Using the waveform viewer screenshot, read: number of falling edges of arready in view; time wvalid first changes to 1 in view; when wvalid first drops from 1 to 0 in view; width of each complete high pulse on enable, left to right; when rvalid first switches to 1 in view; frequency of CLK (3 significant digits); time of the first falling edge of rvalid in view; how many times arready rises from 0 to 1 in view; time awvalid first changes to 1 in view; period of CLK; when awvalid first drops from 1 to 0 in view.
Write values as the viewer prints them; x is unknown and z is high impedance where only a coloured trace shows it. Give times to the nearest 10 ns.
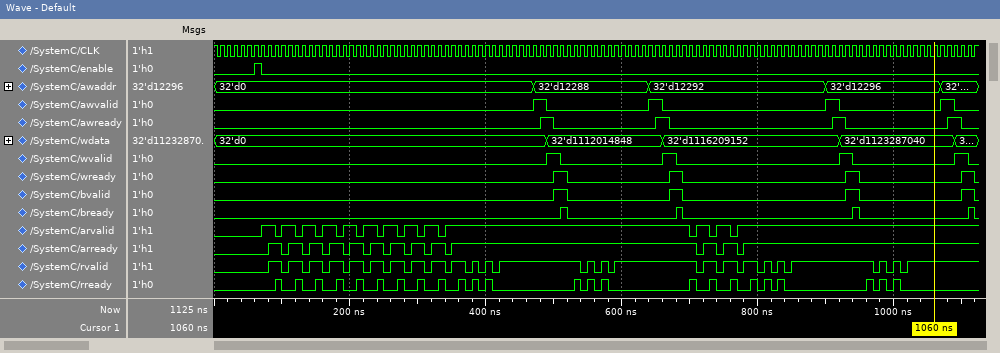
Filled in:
12
490 ns
510 ns
10 ns
80 ns
100 MHz
100 ns
13
470 ns
10 ns
490 ns
